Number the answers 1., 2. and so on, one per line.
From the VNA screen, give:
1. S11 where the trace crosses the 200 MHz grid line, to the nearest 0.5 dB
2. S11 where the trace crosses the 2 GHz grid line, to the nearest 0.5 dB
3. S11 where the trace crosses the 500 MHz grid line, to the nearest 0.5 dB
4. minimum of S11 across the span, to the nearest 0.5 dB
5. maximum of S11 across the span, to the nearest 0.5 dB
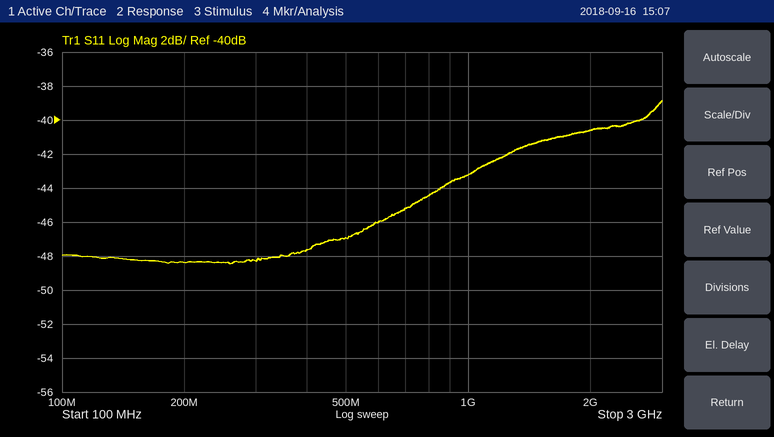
1. -48.5 dB
2. -40.5 dB
3. -47.0 dB
4. -48.5 dB
5. -39.0 dB
